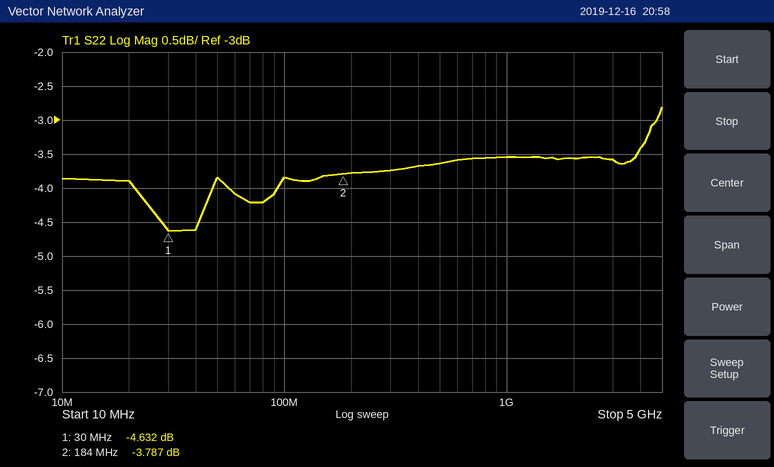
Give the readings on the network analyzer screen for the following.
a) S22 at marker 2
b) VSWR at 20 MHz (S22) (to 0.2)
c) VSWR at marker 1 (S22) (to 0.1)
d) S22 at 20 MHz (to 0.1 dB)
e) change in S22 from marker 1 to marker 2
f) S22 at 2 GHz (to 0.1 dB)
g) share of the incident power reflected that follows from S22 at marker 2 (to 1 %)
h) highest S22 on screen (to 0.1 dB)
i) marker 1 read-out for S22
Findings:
-3.787 dB
4.6
3.8
-3.9 dB
0.845 dB
-3.6 dB
42 %
-2.8 dB
-4.632 dB
